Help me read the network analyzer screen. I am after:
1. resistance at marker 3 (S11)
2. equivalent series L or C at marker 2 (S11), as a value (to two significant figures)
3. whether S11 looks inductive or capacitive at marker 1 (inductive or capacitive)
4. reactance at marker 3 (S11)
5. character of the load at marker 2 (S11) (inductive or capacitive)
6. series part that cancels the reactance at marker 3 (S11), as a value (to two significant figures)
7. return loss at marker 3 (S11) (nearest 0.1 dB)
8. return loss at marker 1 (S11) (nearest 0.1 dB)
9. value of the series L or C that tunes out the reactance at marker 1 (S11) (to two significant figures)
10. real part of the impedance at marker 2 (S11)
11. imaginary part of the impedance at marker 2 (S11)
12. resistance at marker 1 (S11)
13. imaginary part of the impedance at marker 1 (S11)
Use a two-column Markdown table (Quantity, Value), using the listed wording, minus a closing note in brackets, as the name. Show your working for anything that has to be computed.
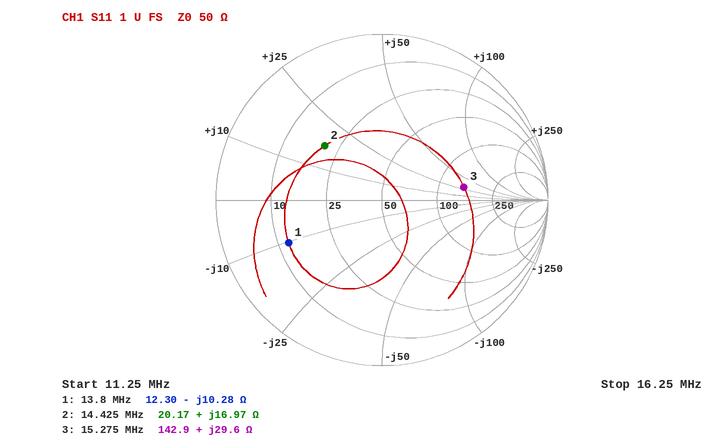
| Quantity | Value |
|---|---|
| resistance at marker 3 | 142.9 Ω |
| equivalent series L or C at marker 2 (S11), as a value | L = 16.97 Ω/(2π × 14.425 MHz) ≈ 187 nH, so 190 nH to two significant figures |
| whether S11 looks inductive or capacitive at marker 1 | capacitive |
| reactance at marker 3 | +29.6 Ω |
| character of the load at marker 2 (S11) | inductive |
| series part that cancels the reactance at marker 3 (S11), as a value | C = 1/(2π × 15.275 MHz × 29.6 Ω) ≈ 352 pF, so 350 pF to two significant figures |
| return loss at marker 3 (S11) | 6.0 dB |
| return loss at marker 1 (S11) | 4.2 dB |
| value of the series L or C that tunes out the reactance at marker 1 (S11) | L = 10.28 Ω/(2π × 13.8 MHz) ≈ 119 nH, so 120 nH to two significant figures |
| real part of the impedance at marker 2 | 20.17 Ω |
| imaginary part of the impedance at marker 2 | +16.97 Ω |
| resistance at marker 1 | 12.30 Ω |
| imaginary part of the impedance at marker 1 | -10.28 Ω |
